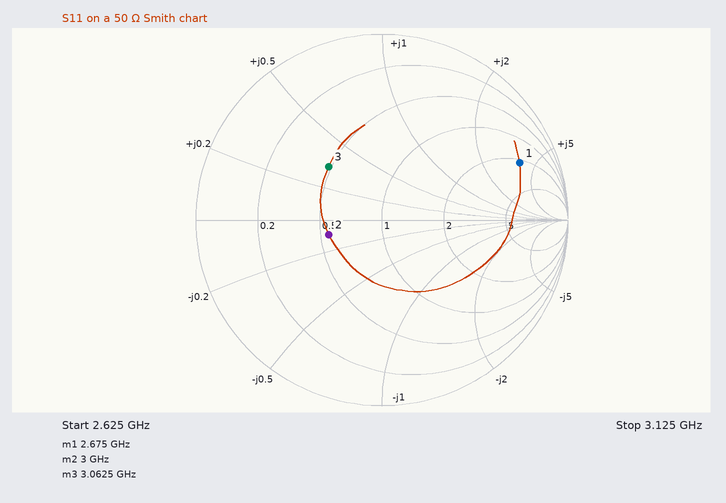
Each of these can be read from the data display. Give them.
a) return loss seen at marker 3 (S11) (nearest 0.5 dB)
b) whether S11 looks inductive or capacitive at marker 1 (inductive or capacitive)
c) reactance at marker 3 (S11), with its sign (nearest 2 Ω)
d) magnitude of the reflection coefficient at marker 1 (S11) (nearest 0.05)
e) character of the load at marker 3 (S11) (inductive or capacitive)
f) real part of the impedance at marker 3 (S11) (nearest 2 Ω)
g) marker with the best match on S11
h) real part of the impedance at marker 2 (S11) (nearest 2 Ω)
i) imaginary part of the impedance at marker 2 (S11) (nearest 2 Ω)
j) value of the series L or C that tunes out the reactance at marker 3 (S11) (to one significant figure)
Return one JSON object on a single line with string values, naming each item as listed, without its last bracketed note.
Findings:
{"return loss seen at marker 3 (S11)": "8.0 dB", "whether S11 looks inductive or capacitive at marker 1": "inductive", "reactance at marker 3 (S11), with its sign": "+16 Ω", "magnitude of the reflection coefficient at marker 1 (S11)": "0.80", "character of the load at marker 3 (S11)": "inductive", "real part of the impedance at marker 3 (S11)": "24 Ω", "marker with the best match on S11": "marker 2", "real part of the impedance at marker 2 (S11)": "28 Ω", "imaginary part of the impedance at marker 2 (S11)": "-4 Ω", "value of the series L or C that tunes out the reactance at marker 3 (S11)": "3 pF"}
